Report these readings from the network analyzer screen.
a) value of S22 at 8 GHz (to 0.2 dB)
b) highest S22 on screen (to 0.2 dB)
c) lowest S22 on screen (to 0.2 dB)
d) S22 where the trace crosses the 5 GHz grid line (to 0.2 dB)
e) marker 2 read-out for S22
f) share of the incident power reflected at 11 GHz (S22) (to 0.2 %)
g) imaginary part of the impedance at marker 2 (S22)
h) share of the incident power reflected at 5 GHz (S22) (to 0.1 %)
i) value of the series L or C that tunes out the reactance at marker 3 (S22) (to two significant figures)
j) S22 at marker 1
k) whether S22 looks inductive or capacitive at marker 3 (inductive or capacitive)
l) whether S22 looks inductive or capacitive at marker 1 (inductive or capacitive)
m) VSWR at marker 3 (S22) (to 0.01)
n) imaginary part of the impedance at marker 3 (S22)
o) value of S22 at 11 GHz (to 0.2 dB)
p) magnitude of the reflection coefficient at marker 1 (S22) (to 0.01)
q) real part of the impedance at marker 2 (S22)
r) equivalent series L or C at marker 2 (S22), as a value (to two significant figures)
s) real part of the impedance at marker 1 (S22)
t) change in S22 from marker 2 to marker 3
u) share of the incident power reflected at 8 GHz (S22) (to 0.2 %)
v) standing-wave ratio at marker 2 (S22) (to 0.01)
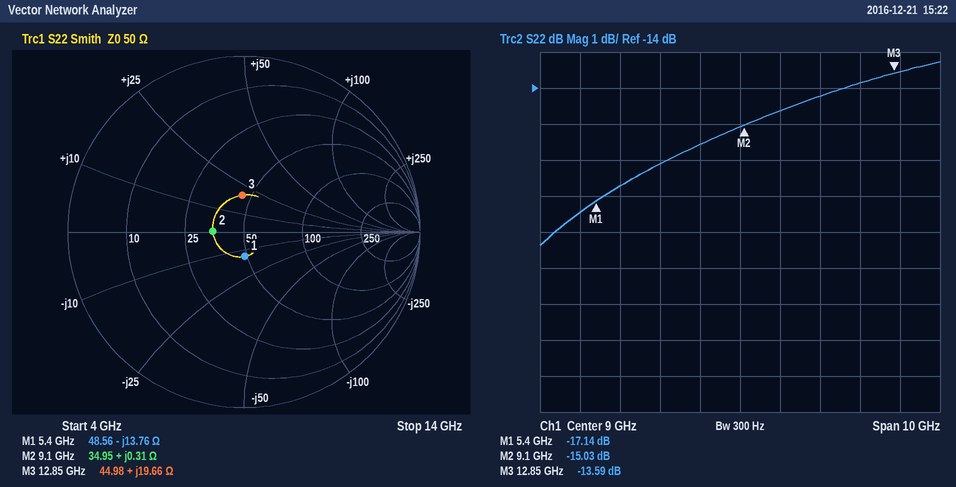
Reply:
-15.6 dB
-13.2 dB
-18.4 dB
-17.4 dB
-15.03 dB
3.8 %
+0.31 Ω
1.8 %
630 fF
-17.14 dB
inductive
capacitive
1.53
+19.66 Ω
-14.2 dB
0.14
34.95 Ω
5.4 pH
48.56 Ω
1.44 dB
2.8 %
1.43
